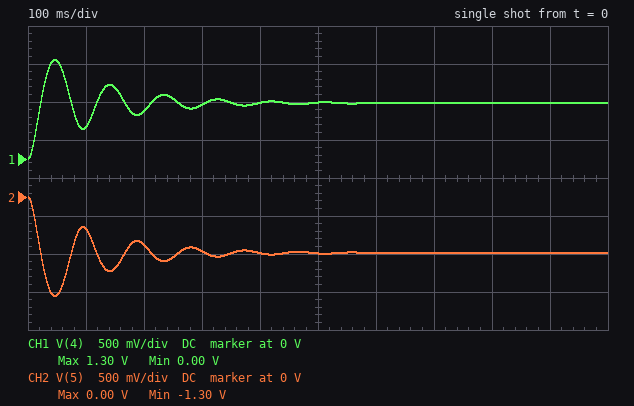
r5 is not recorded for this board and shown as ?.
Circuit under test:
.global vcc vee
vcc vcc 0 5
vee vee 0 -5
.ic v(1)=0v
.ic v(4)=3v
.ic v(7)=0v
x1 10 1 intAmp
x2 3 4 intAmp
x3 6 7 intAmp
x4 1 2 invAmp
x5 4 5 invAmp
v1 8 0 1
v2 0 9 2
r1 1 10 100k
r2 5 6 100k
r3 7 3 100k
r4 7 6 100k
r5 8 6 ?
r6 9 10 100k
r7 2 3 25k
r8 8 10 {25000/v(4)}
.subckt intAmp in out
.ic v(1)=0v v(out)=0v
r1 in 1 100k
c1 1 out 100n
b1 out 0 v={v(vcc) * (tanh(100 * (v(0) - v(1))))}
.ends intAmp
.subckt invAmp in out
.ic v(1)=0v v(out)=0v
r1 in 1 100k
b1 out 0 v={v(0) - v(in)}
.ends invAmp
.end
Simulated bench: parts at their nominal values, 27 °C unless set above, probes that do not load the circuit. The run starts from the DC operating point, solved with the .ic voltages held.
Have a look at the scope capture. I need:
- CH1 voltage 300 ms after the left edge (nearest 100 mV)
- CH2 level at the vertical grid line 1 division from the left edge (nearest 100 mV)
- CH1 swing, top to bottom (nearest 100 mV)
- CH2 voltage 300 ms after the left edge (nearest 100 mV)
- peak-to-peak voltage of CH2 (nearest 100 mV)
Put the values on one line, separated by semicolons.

700 mV; -400 mV; 1.3 V; -700 mV; 1.3 V
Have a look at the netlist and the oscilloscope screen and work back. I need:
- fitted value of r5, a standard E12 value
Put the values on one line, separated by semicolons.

22 kΩ
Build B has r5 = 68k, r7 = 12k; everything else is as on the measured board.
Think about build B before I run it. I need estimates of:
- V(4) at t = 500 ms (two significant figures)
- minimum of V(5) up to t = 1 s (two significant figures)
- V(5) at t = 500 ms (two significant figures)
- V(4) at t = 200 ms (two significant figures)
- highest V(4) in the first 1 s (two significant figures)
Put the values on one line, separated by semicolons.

530 mV; -990 mV; -530 mV; 610 mV; 990 mV
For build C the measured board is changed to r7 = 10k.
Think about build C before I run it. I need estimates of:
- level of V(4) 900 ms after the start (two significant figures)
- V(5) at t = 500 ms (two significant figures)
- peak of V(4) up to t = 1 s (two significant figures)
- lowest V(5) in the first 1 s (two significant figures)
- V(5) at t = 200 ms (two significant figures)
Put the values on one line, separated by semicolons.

600 mV; -600 mV; 1.1 V; -1.1 V; -700 mV
